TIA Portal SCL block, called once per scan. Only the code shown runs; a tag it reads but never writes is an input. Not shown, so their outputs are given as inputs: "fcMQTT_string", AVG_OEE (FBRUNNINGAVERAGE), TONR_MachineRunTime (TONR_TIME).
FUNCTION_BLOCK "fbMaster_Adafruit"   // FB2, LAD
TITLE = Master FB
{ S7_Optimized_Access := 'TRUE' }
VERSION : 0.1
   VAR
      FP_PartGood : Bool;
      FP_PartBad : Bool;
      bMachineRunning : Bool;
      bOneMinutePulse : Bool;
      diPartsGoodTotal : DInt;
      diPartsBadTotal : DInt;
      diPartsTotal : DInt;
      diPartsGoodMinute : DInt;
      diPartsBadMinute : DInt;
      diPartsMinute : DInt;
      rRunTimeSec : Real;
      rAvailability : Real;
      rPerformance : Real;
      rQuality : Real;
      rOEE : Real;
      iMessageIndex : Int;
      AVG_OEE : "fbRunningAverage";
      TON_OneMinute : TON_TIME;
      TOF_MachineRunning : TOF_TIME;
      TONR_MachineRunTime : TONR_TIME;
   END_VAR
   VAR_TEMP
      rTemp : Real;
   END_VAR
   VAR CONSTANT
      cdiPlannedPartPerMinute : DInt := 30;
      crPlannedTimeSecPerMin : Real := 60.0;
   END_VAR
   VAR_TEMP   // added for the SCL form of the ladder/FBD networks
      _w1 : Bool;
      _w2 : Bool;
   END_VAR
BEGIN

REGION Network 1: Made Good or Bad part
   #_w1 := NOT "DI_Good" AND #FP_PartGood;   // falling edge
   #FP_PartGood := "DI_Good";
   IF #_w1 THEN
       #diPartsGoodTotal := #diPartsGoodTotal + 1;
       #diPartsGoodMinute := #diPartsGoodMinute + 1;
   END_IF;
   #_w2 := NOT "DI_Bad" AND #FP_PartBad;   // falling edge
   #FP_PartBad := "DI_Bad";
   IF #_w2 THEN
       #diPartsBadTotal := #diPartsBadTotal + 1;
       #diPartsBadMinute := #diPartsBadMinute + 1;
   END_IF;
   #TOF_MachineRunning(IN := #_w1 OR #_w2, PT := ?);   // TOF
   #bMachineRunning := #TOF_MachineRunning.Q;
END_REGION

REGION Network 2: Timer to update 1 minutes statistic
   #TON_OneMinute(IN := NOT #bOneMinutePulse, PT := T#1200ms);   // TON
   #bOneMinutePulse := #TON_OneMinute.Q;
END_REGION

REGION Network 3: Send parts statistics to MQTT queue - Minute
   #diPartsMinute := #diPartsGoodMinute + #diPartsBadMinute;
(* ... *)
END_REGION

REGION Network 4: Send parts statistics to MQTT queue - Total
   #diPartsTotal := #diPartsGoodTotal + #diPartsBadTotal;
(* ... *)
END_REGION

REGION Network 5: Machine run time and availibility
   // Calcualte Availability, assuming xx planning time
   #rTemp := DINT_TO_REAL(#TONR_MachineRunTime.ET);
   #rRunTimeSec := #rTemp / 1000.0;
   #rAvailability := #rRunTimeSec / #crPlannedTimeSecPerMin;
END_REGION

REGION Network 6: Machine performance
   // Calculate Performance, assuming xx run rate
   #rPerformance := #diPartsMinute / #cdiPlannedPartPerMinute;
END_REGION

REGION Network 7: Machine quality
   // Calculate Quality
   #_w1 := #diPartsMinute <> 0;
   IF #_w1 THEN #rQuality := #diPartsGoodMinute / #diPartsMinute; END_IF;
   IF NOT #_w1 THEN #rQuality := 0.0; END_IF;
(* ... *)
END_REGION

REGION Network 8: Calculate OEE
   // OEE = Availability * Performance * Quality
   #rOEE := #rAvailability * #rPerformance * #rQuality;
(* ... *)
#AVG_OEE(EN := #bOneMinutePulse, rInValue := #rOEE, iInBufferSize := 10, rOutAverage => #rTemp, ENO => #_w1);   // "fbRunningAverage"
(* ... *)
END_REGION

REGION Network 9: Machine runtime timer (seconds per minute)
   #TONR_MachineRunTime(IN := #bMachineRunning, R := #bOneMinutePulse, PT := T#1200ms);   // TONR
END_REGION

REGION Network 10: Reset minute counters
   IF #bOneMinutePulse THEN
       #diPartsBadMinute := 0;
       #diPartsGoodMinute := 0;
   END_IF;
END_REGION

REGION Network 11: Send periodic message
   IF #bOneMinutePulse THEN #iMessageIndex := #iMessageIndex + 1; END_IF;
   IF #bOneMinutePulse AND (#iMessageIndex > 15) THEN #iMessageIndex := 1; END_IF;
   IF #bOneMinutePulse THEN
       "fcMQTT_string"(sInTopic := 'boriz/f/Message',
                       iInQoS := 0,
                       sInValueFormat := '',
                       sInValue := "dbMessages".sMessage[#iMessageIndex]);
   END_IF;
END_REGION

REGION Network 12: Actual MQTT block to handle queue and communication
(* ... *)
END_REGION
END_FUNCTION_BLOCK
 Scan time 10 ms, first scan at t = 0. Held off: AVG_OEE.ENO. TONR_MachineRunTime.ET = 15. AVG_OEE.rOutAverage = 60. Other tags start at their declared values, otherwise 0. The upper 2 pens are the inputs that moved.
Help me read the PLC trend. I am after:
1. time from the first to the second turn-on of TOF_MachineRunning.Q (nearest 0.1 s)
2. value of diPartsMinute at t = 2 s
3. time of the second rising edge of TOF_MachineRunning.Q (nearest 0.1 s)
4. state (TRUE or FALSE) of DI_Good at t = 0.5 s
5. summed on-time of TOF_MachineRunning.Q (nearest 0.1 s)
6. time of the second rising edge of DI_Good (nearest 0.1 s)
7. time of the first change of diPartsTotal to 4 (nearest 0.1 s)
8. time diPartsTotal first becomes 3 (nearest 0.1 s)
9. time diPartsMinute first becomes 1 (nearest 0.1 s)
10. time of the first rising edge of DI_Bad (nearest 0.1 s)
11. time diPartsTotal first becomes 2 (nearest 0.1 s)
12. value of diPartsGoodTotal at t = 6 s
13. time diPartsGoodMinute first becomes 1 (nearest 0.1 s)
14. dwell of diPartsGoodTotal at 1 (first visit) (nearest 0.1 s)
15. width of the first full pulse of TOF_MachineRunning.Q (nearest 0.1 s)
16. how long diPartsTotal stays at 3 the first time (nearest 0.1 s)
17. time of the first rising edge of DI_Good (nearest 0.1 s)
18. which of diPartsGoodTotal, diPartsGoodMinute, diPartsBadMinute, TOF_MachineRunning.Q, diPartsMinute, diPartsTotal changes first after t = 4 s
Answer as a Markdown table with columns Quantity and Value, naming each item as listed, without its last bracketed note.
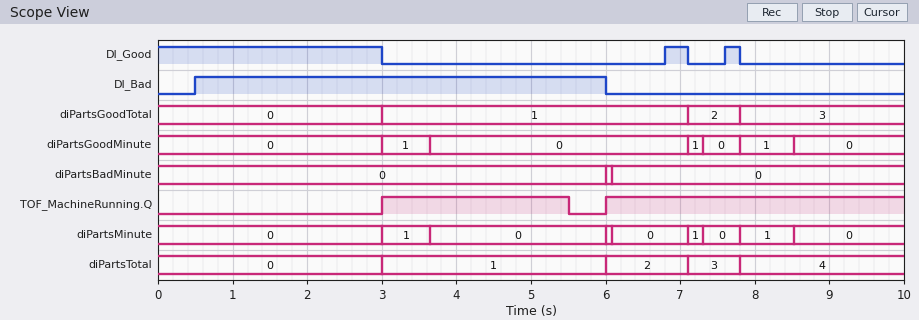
| Quantity | Value |
|---|---|
| time from the first to the second turn-on of TOF_MachineRunning.Q | 3.0 s |
| value of diPartsMinute at t = 2 s | 0 |
| time of the second rising edge of TOF_MachineRunning.Q | 6.0 s |
| state (TRUE or FALSE) of DI_Good at t = 0.5 s | TRUE |
| summed on-time of TOF_MachineRunning.Q | 6.5 s |
| time of the second rising edge of DI_Good | 7.6 s |
| time of the first change of diPartsTotal to 4 | 7.8 s |
| time diPartsTotal first becomes 3 | 7.1 s |
| time diPartsMinute first becomes 1 | 3.0 s |
| time of the first rising edge of DI_Bad | 0.5 s |
| time diPartsTotal first becomes 2 | 6.0 s |
| value of diPartsGoodTotal at t = 6 s | 1 |
| time diPartsGoodMinute first becomes 1 | 3.0 s |
| dwell of diPartsGoodTotal at 1 (first visit) | 4.1 s |
| width of the first full pulse of TOF_MachineRunning.Q | 2.5 s |
| how long diPartsTotal stays at 3 the first time | 0.7 s |
| time of the first rising edge of DI_Good | 6.8 s |
| which of diPartsGoodTotal, diPartsGoodMinute, diPartsBadMinute, TOF_MachineRunning.Q, diPartsMinute, diPartsTotal changes first after t = 4 s | TOF_MachineRunning.Q |
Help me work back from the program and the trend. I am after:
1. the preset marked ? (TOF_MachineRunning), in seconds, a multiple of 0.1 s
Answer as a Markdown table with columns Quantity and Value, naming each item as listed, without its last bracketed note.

| Quantity | Value |
|---|---|
| the preset marked ? (TOF_MachineRunning), in seconds, a multiple of 0.1 s | 2.5 s |
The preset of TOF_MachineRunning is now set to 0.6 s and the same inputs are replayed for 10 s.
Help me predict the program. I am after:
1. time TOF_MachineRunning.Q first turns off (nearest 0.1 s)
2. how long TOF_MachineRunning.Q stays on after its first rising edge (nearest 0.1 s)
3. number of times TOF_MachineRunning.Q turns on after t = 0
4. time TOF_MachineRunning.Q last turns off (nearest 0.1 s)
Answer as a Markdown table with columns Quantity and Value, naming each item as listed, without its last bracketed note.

| Quantity | Value |
|---|---|
| time TOF_MachineRunning.Q first turns off | 3.6 s |
| how long TOF_MachineRunning.Q stays on after its first rising edge | 0.6 s |
| number of times TOF_MachineRunning.Q turns on after t = 0 | 4 |
| time TOF_MachineRunning.Q last turns off | 8.4 s |
